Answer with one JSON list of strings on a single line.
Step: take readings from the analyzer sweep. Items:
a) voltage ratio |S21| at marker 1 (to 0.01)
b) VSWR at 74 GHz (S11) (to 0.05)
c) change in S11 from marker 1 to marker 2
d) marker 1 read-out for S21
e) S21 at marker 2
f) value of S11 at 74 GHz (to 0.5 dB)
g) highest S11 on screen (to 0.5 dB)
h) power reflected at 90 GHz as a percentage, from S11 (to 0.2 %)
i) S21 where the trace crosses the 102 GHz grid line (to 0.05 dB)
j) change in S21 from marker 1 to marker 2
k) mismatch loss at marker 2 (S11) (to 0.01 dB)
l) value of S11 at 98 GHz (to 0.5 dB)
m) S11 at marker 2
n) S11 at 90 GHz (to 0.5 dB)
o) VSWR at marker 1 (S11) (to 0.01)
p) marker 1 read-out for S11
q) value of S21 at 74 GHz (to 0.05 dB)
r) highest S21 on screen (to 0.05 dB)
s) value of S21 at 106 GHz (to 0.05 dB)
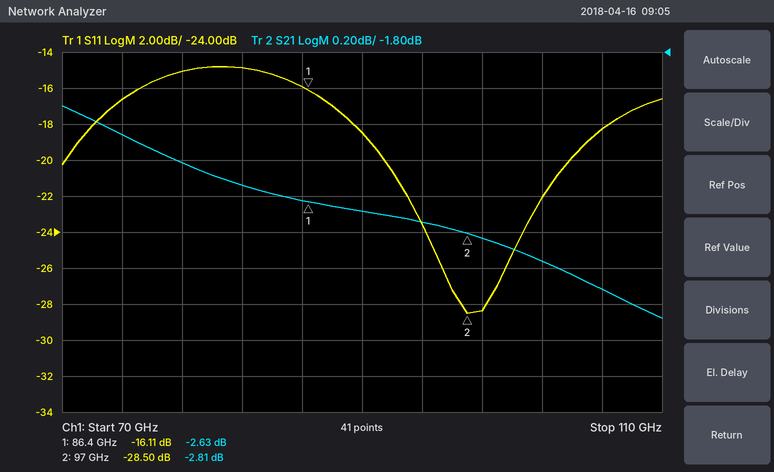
["0.74", "1.35", "-12.39 dB", "-2.63 dB", "-2.81 dB", "-16.5 dB", "-15.0 dB", "1.4 %", "-2.95 dB", "-0.18 dB", "0.01 dB", "-28.5 dB", "-28.50 dB", "-18.5 dB", "1.37", "-16.11 dB", "-2.25 dB", "-2.10 dB", "-3.10 dB"]
